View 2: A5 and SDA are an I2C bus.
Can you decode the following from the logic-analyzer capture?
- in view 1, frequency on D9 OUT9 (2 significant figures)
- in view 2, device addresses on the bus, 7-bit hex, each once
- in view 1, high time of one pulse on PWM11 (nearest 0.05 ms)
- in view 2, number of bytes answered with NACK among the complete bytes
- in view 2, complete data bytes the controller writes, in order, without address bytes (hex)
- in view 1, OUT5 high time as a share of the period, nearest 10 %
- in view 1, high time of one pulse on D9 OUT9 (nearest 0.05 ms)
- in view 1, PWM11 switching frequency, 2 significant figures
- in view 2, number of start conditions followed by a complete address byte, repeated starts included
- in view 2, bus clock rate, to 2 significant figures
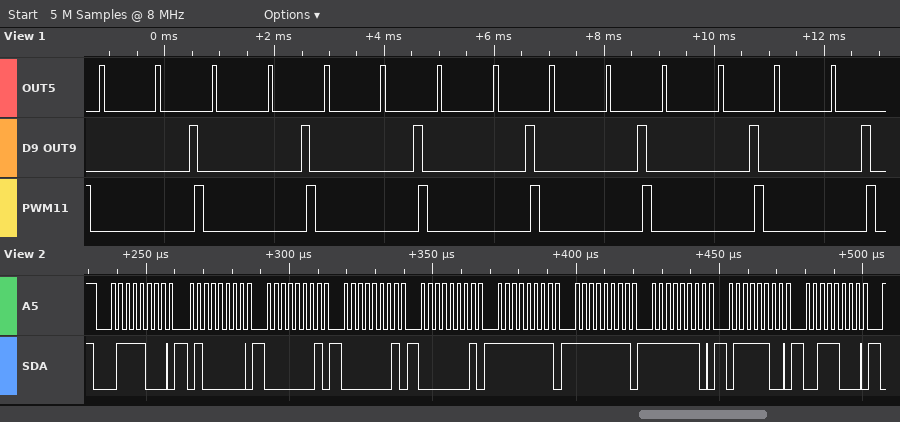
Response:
490 Hz
0x3C
0.15 ms
0
40 01 01 01 FF FF FE 7C 38
10 %
0.15 ms
490 Hz
1
400 kHz
